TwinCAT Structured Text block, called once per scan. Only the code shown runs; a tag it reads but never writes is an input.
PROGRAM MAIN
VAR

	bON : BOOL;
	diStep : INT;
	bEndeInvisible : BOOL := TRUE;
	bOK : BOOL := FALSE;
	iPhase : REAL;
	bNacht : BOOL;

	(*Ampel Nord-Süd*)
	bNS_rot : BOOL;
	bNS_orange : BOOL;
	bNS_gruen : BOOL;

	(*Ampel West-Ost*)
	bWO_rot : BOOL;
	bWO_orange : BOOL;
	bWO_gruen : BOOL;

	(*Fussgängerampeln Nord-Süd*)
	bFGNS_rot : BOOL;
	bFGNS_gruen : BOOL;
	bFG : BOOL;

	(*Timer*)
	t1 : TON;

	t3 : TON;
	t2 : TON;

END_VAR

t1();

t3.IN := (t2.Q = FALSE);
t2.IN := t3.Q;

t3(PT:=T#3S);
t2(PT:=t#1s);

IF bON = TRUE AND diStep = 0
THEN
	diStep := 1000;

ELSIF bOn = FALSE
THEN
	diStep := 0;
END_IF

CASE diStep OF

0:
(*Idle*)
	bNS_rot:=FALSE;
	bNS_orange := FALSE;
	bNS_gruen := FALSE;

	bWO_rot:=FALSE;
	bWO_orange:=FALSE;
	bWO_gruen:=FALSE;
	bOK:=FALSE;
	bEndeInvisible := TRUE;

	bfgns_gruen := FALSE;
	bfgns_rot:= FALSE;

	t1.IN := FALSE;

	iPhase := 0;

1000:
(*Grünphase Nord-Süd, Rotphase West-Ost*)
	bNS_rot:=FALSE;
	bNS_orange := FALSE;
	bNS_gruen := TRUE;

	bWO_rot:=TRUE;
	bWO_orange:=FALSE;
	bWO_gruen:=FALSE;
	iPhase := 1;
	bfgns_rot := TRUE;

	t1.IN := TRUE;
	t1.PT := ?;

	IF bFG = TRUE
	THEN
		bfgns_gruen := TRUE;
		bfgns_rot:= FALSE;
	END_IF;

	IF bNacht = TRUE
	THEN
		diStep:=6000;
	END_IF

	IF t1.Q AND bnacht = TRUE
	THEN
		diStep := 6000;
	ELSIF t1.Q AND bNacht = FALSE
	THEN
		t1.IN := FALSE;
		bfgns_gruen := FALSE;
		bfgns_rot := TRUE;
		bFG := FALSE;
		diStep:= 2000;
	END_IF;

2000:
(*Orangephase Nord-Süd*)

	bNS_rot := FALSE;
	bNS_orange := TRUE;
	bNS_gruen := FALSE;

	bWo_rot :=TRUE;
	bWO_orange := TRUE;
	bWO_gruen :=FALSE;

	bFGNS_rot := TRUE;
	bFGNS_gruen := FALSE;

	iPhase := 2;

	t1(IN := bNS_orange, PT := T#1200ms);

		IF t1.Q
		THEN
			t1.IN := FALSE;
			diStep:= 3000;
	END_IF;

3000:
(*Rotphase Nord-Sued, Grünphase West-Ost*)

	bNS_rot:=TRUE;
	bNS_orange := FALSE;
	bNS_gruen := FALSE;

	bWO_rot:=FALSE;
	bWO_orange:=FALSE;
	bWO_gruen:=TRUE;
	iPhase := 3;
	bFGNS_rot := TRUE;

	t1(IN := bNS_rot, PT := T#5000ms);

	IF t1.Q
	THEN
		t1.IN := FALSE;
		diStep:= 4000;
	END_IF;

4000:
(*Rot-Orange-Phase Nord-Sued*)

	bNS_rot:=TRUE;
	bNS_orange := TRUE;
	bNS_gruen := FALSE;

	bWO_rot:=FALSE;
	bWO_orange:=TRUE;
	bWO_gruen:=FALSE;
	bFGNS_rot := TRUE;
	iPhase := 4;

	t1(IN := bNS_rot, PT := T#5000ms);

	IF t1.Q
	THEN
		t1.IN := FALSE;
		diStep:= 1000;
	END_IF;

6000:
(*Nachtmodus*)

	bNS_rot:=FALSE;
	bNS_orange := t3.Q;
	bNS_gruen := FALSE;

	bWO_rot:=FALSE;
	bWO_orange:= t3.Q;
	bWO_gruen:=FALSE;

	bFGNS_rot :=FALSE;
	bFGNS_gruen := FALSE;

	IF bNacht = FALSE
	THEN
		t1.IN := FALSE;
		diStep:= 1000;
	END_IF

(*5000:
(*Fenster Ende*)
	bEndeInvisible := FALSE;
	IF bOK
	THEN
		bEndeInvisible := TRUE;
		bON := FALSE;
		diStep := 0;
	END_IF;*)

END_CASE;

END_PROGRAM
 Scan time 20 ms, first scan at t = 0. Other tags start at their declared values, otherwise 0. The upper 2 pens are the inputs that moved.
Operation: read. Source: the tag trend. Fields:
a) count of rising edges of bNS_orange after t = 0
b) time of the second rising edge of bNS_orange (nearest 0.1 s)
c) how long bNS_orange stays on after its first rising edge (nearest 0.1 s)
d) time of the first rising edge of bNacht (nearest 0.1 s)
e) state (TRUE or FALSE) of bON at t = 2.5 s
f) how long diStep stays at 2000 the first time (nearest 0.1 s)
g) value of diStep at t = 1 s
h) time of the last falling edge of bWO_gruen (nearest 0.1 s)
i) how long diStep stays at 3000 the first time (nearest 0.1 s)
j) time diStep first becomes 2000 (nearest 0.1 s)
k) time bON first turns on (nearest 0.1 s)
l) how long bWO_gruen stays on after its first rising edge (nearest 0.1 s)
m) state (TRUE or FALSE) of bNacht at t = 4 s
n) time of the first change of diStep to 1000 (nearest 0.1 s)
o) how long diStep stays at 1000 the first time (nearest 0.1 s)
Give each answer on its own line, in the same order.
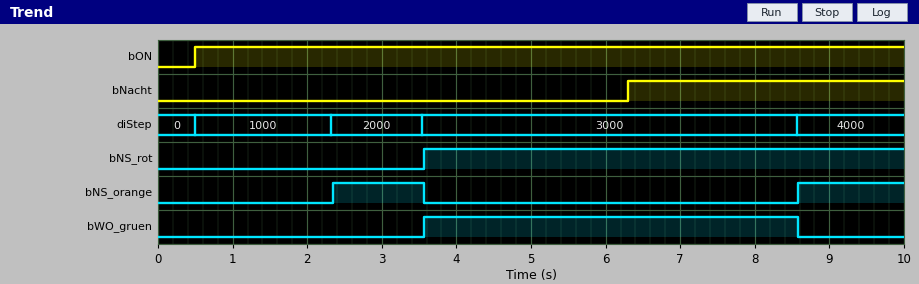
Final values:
2
8.6 s
1.2 s
6.3 s
TRUE
1.2 s
1000
8.6 s
5.0 s
2.3 s
0.5 s
5.0 s
FALSE
0.5 s
1.8 s
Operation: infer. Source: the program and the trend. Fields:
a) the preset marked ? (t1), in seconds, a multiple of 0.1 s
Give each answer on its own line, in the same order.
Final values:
1.8 s
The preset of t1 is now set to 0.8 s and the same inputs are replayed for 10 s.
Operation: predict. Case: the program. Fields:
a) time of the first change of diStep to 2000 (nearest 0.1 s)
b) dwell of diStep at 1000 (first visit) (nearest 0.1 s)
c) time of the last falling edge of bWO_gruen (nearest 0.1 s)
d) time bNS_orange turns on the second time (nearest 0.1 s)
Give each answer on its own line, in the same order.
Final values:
1.3 s
0.8 s
7.6 s
7.6 s
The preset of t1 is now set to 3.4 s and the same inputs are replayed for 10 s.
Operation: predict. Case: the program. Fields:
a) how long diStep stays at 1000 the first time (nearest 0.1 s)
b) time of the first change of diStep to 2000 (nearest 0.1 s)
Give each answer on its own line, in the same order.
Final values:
3.4 s
3.9 s
